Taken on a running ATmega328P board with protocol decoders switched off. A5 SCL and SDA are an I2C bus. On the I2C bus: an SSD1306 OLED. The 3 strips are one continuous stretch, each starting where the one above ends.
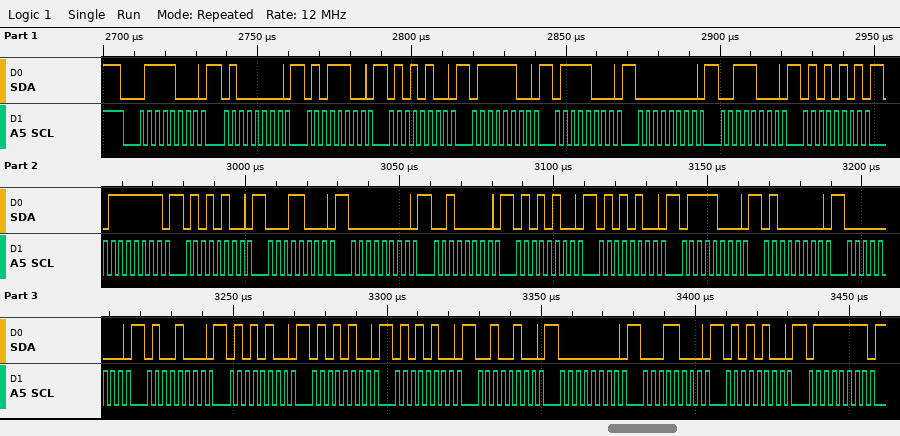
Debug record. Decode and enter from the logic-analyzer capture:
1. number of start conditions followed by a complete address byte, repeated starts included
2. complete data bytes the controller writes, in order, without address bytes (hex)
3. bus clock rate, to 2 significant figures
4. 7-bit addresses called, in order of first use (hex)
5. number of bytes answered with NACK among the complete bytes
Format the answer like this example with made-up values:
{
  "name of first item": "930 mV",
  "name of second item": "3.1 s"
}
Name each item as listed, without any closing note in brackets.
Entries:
{
  "number of start conditions followed by a complete address byte, repeated starts included": "1",
  "complete data bytes the controller writes, in order, without address bytes": "40 5C 54 7C 78 00 38 55 7F 54 18 00 20 54 54 78 40 00 48 54 54 54 24 00 18 54 7F",
  "bus clock rate, to 2 significant figures": "400 kHz",
  "7-bit addresses called, in order of first use": "0x3C",
  "number of bytes answered with NACK among the complete bytes": "0"
}
